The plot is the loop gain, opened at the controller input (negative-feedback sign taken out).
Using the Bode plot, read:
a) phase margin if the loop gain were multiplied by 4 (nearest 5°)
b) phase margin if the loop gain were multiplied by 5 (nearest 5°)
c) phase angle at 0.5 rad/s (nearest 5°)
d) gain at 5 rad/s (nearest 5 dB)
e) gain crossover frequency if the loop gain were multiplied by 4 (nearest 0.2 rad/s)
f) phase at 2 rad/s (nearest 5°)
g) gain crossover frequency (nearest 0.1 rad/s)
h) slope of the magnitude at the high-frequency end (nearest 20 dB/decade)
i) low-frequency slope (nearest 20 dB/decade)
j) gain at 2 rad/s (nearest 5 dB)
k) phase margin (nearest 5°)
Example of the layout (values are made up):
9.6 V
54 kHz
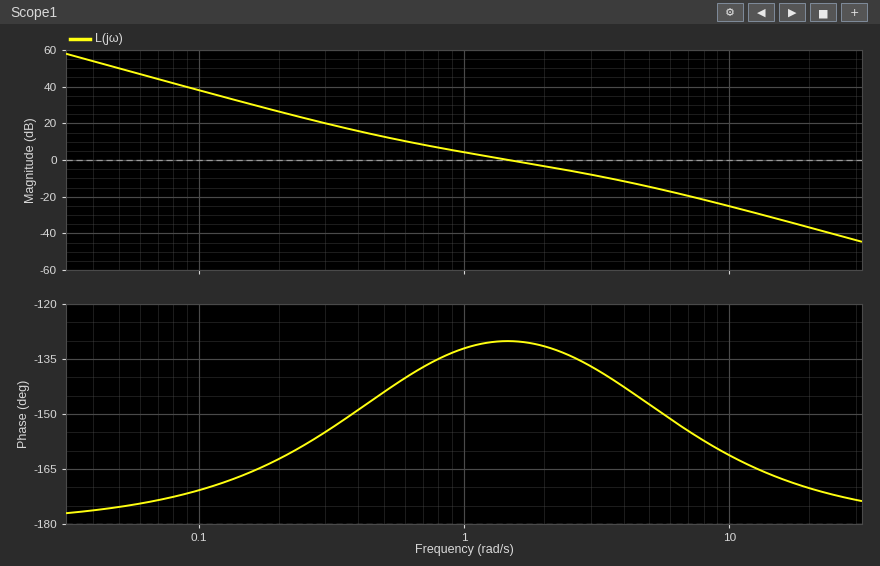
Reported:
35°
35°
-145°
-15 dB
4.2 rad/s
-130°
1.5 rad/s
-40 dB/decade
-40 dB/decade
-5 dB
50°
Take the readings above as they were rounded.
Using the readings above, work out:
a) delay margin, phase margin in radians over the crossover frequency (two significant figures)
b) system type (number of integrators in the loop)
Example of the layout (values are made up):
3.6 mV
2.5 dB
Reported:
0.58 s
2
